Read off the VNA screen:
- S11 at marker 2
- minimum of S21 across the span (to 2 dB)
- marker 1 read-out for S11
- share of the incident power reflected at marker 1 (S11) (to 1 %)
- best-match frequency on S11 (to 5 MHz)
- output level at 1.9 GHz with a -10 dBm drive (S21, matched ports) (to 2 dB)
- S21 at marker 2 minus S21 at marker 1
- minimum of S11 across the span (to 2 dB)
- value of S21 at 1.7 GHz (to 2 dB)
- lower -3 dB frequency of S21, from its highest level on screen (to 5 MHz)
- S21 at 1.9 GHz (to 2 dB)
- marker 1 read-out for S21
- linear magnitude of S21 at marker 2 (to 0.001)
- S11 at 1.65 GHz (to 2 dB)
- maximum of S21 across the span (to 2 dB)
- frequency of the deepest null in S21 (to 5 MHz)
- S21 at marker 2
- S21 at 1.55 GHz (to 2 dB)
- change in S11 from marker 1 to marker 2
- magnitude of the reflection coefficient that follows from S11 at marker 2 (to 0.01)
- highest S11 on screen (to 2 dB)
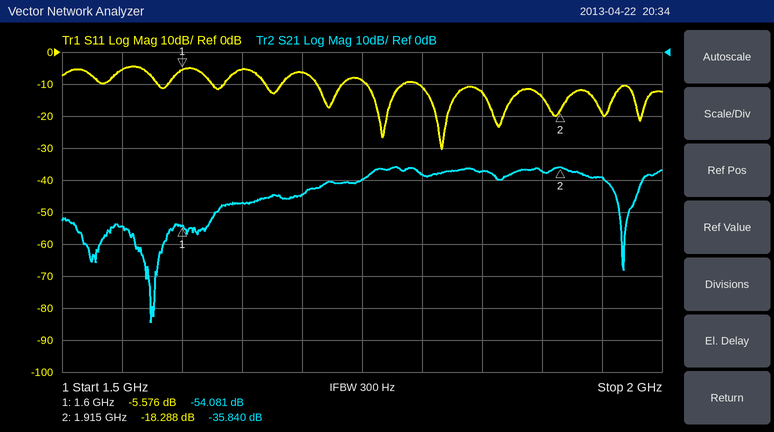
-18.288 dB
-84 dB
-5.576 dB
28 %
1.815 GHz
-48 dBm
18.241 dB
-30 dB
-44 dB
1.755 GHz
-38 dB
-54.081 dB
0.016
-6 dB
-36 dB
1.575 GHz
-35.840 dB
-54 dB
-12.712 dB
0.12
-4 dB
